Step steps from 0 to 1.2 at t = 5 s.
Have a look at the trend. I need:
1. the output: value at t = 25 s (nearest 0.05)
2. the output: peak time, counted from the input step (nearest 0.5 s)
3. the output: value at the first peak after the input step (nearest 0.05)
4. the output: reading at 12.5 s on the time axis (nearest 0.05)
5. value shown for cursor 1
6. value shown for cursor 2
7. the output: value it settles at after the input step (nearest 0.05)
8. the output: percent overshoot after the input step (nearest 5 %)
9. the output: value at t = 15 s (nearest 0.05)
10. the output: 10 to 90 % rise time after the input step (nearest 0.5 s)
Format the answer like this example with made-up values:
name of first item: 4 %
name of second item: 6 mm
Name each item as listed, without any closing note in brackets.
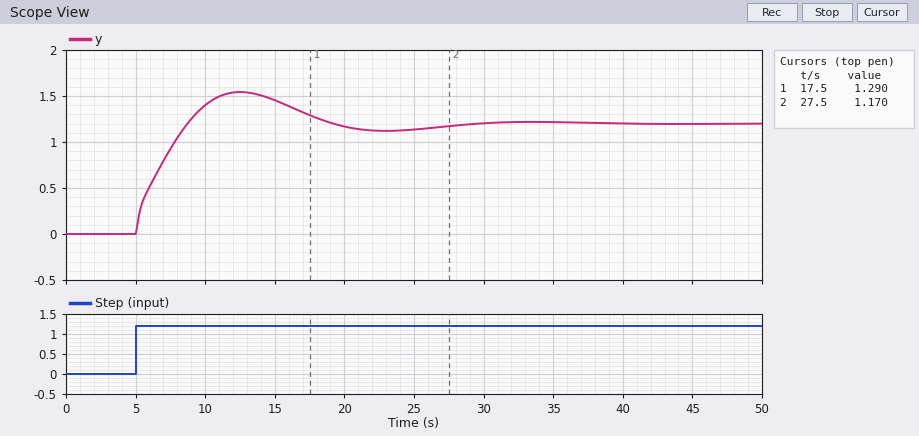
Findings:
the output: value at t = 25 s: 1.15
the output: peak time, counted from the input step: 7.5 s
the output: value at the first peak after the input step: 1.55
the output: reading at 12.5 s on the time axis: 1.55
value shown for cursor 1: 1.290
value shown for cursor 2: 1.170
the output: value it settles at after the input step: 1.20
the output: percent overshoot after the input step: 30 %
the output: value at t = 15 s: 1.45
the output: 10 to 90 % rise time after the input step: 3.0 s
